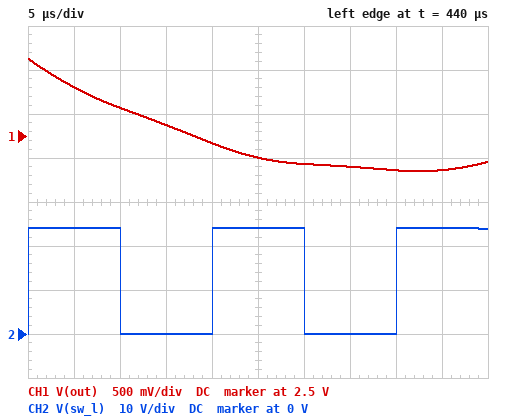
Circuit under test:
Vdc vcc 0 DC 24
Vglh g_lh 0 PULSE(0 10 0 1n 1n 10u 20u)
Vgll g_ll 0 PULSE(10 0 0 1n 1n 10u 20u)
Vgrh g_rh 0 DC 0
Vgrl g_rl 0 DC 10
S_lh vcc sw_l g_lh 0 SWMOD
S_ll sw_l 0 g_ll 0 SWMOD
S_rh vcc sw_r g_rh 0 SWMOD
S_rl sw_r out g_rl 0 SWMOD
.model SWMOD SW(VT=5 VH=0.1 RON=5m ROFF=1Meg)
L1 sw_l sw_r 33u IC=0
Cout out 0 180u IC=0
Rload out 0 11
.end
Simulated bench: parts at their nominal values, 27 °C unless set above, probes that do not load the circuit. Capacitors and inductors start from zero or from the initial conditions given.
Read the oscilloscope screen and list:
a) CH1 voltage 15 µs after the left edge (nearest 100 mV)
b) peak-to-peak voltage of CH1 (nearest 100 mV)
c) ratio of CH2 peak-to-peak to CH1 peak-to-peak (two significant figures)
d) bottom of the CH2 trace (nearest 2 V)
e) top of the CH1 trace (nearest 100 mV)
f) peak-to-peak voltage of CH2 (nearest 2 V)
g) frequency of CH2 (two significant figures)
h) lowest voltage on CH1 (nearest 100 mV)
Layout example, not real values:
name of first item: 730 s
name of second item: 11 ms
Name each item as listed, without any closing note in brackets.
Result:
CH1 voltage 15 µs after the left edge: 2.6 V
peak-to-peak voltage of CH1: 1.3 V
ratio of CH2 peak-to-peak to CH1 peak-to-peak: 19
bottom of the CH2 trace: 0 V
top of the CH1 trace: 3.4 V
peak-to-peak voltage of CH2: 24 V
frequency of CH2: 50 kHz
lowest voltage on CH1: 2.1 V
